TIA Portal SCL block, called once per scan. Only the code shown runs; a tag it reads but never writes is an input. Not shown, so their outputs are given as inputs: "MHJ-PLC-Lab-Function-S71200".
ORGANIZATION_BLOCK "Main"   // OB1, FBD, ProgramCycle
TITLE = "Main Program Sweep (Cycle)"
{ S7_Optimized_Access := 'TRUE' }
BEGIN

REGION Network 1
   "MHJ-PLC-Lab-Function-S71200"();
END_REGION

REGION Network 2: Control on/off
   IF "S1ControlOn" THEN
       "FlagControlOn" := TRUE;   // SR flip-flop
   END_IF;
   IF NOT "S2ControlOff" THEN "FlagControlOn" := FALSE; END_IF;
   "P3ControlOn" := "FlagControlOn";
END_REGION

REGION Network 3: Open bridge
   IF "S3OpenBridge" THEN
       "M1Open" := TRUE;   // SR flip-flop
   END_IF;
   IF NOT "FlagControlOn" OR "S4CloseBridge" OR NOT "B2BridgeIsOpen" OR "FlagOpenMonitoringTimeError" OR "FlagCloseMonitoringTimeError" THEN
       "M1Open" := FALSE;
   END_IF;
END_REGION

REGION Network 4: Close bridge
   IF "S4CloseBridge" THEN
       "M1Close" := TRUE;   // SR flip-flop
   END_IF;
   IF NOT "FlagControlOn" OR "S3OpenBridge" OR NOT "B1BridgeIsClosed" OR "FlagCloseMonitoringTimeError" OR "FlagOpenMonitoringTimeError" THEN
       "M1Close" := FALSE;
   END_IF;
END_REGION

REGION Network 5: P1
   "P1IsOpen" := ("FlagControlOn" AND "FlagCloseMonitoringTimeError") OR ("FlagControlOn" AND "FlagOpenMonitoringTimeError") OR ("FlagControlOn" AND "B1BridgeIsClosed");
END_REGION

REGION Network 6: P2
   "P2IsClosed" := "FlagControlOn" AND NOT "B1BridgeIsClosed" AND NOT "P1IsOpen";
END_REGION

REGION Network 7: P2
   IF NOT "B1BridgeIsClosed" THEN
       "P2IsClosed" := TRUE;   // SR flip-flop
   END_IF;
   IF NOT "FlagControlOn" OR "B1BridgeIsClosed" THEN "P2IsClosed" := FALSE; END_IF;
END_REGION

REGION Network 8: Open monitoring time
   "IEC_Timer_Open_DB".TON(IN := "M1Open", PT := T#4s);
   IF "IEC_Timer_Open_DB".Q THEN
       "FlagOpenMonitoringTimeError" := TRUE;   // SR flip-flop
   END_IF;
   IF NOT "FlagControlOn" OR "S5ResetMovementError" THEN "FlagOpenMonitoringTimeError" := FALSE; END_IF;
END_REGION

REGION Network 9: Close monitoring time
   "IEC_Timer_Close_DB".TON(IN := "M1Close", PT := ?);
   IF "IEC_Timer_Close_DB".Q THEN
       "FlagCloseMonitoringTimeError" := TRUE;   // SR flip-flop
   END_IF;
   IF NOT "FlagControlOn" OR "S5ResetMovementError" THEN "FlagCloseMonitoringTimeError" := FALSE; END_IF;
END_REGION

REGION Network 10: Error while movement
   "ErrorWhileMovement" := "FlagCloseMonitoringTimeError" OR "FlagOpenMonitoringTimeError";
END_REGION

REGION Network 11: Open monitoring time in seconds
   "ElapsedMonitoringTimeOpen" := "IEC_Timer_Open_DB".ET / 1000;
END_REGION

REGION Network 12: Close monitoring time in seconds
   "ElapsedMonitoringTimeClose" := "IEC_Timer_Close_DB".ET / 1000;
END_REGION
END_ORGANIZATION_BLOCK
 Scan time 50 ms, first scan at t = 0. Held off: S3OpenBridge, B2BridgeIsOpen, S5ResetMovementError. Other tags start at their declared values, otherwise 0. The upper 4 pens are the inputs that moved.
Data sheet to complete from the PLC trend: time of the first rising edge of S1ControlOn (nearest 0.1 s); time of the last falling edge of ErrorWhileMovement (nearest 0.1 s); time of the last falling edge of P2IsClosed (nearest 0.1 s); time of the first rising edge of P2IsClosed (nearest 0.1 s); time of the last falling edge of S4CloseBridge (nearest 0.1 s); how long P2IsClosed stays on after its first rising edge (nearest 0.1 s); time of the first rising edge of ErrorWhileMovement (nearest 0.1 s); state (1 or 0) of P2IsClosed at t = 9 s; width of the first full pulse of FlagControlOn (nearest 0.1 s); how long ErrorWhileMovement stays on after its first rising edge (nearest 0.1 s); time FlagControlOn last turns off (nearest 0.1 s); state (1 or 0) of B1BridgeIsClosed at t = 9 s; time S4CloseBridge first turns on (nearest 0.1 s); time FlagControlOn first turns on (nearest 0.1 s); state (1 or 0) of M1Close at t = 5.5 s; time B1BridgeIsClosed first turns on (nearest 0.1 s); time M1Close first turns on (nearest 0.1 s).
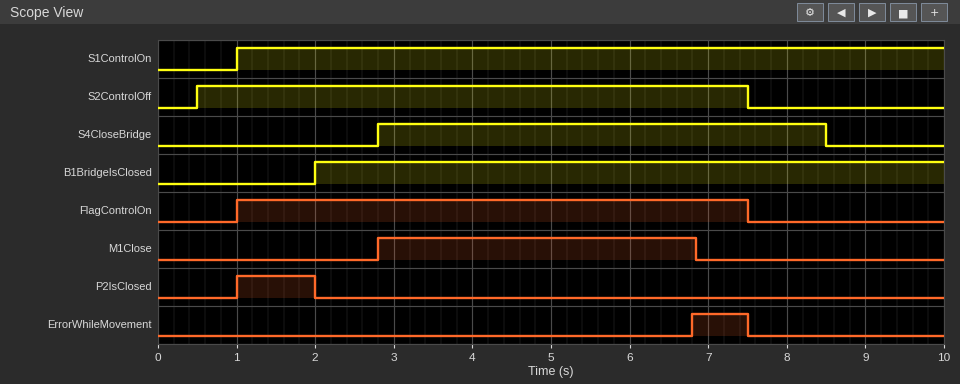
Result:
1.0 s
7.5 s
2.0 s
1.0 s
8.5 s
1.0 s
6.8 s
0
6.5 s
0.7 s
7.5 s
1
2.8 s
1.0 s
1
2.0 s
2.8 s
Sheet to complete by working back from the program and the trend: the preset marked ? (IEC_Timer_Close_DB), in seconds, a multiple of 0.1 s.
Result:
4.0 s
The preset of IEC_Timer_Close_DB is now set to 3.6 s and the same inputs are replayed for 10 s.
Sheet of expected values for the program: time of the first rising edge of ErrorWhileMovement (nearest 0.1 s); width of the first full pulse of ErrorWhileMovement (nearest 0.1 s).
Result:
6.4 s
1.1 s
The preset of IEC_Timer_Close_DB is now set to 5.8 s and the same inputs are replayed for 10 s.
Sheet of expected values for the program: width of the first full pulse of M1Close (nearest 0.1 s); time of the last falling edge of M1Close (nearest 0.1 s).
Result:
4.7 s
7.5 s
